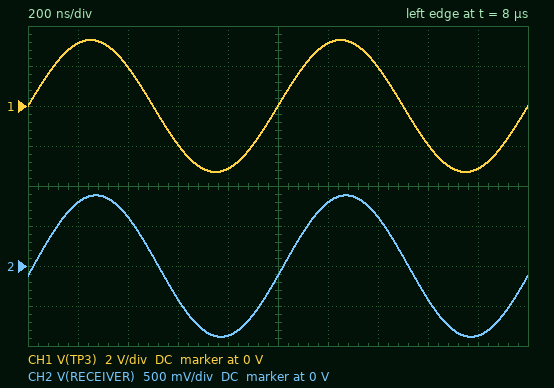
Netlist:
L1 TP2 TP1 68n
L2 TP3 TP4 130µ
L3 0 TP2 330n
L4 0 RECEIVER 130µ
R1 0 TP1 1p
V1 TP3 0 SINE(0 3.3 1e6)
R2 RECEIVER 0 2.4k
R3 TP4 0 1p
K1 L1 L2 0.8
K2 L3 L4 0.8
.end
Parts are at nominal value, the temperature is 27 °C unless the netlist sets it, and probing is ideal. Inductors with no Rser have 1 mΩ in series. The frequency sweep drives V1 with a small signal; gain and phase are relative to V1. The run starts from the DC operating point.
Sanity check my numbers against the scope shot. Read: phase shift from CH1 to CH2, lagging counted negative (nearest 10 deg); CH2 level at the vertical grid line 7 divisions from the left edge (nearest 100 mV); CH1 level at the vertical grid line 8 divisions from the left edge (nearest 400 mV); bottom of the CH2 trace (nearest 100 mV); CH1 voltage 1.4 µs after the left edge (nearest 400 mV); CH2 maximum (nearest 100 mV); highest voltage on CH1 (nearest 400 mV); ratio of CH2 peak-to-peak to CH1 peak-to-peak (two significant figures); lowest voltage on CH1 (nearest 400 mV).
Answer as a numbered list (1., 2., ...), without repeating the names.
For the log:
1. -10 deg
2. 600 mV
3. -2.0 V
4. -900 mV
5. 2.0 V
6. 900 mV
7. 3.2 V
8. 0.27
9. -3.2 V
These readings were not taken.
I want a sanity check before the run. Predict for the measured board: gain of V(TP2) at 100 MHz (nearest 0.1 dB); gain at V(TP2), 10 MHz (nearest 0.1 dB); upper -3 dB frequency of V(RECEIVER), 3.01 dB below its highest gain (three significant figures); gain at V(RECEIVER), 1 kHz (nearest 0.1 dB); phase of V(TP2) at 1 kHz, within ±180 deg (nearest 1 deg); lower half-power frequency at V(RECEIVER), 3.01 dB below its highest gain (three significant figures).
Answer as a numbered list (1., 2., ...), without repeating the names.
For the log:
1. -36.4 dB
2. -36.0 dB
3. 7.27 MHz
4. -13.9 dB
5. 16 deg
6. 898 Hz
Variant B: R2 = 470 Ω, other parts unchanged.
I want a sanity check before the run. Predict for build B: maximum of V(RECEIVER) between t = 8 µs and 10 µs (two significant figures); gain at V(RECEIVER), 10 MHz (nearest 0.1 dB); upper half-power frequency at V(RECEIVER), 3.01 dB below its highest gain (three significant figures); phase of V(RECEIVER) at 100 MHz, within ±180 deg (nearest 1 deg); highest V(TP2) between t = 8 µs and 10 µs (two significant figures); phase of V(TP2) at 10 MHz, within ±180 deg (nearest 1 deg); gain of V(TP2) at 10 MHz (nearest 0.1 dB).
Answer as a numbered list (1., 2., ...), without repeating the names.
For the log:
1. 730 mV
2. -28.4 dB
3. 1.43 MHz
4. -89 deg
5. 54 mV
6. -1 deg
7. -36.4 dB
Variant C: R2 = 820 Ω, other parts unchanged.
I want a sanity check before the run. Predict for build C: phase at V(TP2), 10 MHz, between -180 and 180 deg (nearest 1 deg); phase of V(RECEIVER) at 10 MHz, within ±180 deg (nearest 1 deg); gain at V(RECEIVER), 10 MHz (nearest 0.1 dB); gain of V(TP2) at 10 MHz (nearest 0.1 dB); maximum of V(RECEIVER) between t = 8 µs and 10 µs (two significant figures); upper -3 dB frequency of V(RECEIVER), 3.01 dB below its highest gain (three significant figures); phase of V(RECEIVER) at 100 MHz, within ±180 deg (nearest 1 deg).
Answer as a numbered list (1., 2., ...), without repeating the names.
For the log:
1. -2 deg
2. -76 deg
3. -23.7 dB
4. -36.3 dB
5. 830 mV
6. 2.49 MHz
7. -89 deg
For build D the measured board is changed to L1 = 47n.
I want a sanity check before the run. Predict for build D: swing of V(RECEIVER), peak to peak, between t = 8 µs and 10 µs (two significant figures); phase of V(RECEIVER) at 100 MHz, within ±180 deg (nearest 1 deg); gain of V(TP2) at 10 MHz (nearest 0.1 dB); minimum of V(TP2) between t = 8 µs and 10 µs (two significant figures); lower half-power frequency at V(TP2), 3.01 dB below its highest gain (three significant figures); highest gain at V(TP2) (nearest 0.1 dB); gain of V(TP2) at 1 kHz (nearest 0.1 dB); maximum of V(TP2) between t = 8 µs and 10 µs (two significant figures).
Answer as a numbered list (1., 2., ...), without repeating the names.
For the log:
1. 1.5 V
2. -86 deg
3. -37.2 dB
4. -48 mV
5. 614 Hz
6. -36.8 dB
7. -38.5 dB
8. 48 mV
